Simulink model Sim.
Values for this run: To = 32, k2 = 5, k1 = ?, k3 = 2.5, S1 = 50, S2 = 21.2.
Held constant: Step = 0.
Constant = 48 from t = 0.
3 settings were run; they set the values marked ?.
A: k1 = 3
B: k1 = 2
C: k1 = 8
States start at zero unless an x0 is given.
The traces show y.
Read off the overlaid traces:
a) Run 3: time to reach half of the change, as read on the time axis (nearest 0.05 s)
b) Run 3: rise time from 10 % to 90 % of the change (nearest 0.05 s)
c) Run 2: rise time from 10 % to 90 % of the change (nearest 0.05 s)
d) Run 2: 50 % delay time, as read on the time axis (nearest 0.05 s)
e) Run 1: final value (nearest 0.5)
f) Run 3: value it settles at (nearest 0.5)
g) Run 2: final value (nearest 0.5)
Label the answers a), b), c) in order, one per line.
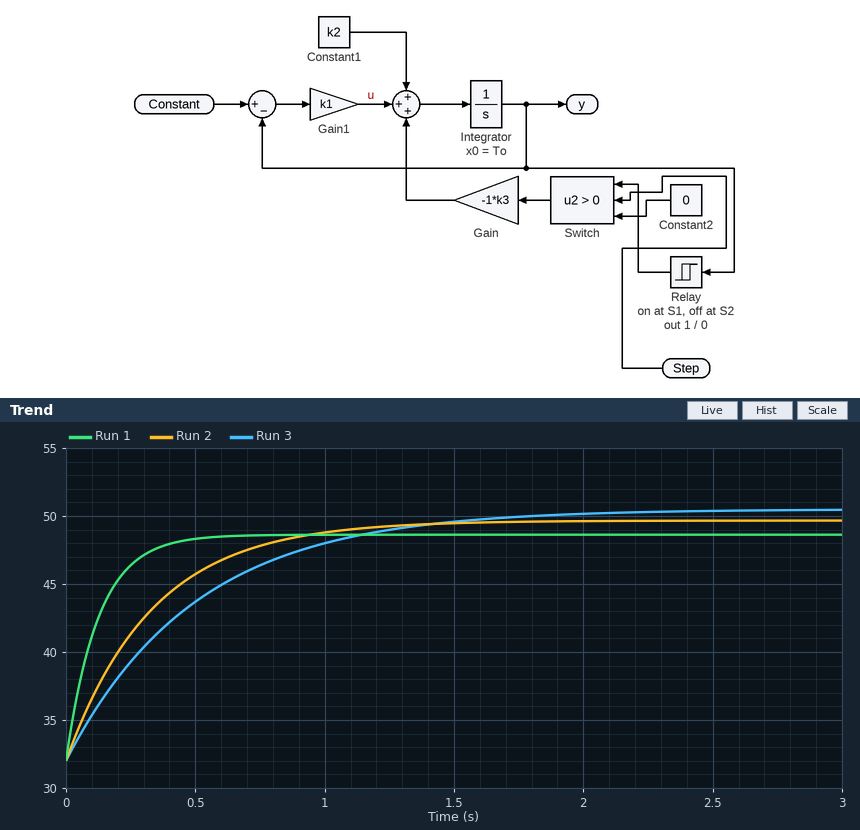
a) 0.35 s
b) 1.10 s
c) 0.75 s
d) 0.25 s
e) 48.5
f) 50.5
g) 49.5
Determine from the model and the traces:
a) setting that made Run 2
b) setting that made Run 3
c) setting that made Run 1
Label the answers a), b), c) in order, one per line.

a) A
b) B
c) C
